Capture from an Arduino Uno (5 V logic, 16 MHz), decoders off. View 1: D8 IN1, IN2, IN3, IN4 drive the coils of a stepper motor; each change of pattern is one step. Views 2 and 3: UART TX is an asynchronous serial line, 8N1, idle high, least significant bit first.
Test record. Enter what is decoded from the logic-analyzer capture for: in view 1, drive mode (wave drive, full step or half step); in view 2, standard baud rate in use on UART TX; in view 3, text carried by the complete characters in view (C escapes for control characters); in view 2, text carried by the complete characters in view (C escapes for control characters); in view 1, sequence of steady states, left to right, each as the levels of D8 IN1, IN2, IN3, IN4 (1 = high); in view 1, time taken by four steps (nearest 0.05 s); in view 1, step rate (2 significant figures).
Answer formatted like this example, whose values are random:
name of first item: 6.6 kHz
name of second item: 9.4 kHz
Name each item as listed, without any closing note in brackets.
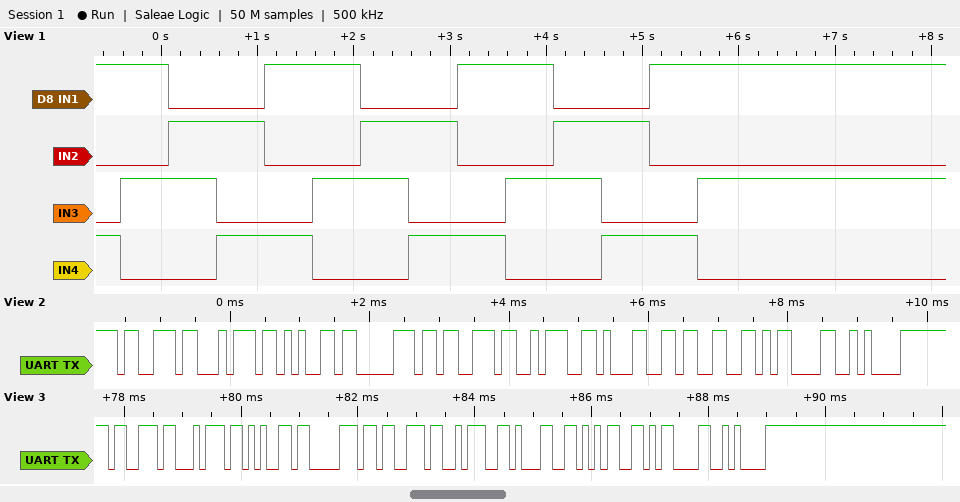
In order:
in view 1, drive mode: full step
in view 2, standard baud rate in use on UART TX: 9600 baud
in view 3, text carried by the complete characters in view: "steps:15\r\n"
in view 2, text carried by the complete characters in view: "steps:13\r\n"
in view 1, sequence of steady states, left to right, each as the levels of D8 IN1, IN2, IN3, IN4: 1001 1010 0110 0101 1001 1010 0110 0101 1001 1010 0110 0101 1001 1010
in view 1, time taken by four steps: 2.00 s
in view 1, step rate: 2.0 steps/s
